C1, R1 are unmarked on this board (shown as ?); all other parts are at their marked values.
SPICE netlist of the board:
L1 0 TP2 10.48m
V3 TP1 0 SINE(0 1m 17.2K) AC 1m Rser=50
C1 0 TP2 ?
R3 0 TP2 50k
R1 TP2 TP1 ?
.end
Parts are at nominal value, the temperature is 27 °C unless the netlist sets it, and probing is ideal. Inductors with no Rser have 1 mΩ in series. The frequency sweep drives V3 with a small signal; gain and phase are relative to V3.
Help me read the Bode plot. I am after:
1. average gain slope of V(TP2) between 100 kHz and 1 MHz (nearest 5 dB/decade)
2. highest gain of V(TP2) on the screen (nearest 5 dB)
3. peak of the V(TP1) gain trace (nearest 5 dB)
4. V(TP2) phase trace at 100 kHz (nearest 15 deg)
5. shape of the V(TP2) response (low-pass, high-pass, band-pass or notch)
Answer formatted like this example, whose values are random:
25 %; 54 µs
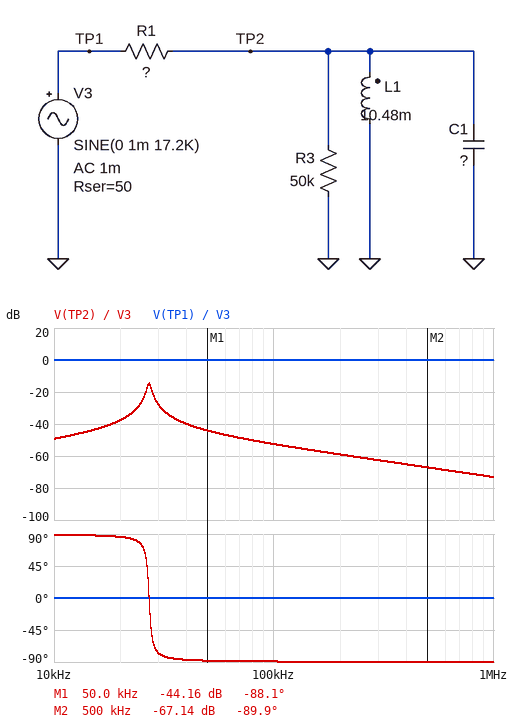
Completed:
-20 dB/decade; -15 dB; 0 dB; -90 deg; band-pass
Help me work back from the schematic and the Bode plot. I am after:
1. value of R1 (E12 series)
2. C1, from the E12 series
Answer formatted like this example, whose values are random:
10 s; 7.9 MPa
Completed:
220 kΩ; 3.3 nF
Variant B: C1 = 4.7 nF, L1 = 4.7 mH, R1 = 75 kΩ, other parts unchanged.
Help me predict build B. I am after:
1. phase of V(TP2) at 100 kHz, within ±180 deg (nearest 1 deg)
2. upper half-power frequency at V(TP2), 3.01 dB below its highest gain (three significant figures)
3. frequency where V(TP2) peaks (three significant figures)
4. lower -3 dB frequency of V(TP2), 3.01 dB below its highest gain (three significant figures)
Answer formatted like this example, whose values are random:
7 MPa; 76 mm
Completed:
-89 deg; 34.4 kHz; 33.9 kHz; 33.3 kHz
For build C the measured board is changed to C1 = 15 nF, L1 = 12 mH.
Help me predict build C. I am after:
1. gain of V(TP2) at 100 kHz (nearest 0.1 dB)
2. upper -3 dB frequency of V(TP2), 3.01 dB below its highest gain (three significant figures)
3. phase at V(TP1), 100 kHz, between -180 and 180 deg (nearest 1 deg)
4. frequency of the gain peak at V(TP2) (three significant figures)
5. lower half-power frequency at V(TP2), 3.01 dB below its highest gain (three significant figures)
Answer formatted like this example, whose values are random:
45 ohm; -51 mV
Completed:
-66.2 dB; 12.0 kHz; 0 deg; 11.9 kHz; 11.7 kHz
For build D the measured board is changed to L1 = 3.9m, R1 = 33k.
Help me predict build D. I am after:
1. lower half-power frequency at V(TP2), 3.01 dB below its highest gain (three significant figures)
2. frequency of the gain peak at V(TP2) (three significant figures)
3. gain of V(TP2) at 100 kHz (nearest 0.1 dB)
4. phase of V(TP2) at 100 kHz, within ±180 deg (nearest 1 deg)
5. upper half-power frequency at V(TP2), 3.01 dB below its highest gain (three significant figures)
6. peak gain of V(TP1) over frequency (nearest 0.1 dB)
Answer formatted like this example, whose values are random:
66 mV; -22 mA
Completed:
43.2 kHz; 44.4 kHz; -34.8 dB; -88 deg; 45.6 kHz; 0 dB
